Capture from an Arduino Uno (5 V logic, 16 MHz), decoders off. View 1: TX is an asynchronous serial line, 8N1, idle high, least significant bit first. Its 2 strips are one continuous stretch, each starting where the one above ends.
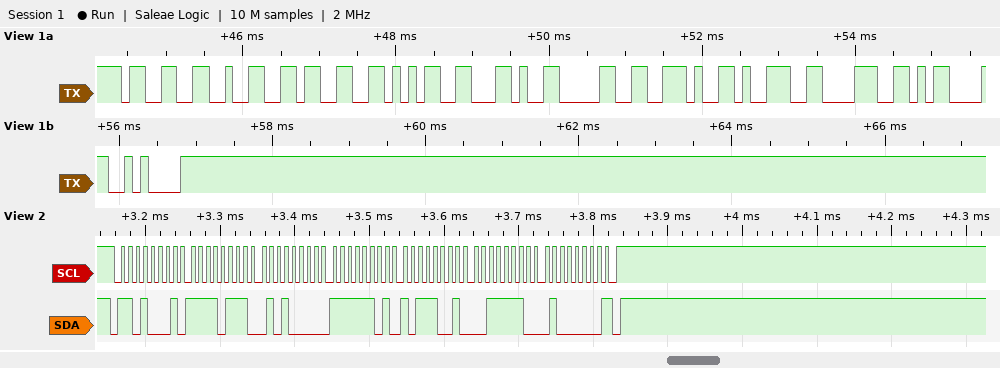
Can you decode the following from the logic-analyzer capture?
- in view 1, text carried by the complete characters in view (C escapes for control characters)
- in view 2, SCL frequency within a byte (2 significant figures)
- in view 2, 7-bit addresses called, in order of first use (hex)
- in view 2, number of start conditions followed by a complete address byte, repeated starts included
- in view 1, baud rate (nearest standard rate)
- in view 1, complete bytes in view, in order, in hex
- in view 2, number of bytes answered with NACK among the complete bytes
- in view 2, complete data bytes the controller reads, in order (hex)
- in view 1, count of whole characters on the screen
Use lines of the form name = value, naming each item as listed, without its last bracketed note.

in view 1, text carried by the complete characters in view = "3235,0.98\r\n"
in view 2, SCL frequency within a byte = 100 kHz
in view 2, 7-bit addresses called, in order of first use = 0x68
in view 2, number of start conditions followed by a complete address byte, repeated starts included = 1
in view 1, baud rate = 9600 baud
in view 1, complete bytes in view, in order, in hex = 33 32 33 35 2C 30 2E 39 38 0D 0A
in view 2, number of bytes answered with NACK among the complete bytes = 1
in view 2, complete data bytes the controller reads, in order = F7 50 FD B9 3E 40
in view 1, count of whole characters on the screen = 11
